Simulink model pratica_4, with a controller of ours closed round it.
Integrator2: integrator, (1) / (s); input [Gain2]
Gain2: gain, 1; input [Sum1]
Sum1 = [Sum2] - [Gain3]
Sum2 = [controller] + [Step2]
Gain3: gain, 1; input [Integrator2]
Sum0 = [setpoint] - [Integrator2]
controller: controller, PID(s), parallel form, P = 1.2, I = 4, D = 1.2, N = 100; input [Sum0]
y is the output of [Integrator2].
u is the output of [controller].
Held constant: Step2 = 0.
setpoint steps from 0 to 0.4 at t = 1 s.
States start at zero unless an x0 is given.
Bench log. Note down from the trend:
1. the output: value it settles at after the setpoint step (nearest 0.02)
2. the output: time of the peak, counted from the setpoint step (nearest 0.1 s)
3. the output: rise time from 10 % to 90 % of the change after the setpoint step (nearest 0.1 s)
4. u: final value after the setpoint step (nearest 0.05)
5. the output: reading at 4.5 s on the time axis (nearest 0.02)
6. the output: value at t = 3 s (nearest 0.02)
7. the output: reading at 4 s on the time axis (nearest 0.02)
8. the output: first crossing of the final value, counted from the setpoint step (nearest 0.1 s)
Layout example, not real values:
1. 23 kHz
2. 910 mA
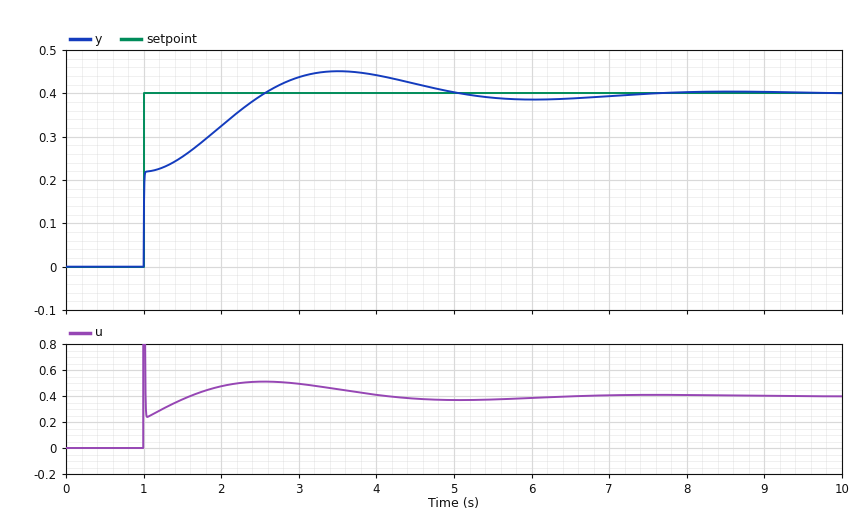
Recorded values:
1. 0.40
2. 2.5 s
3. 1.2 s
4. 0.40
5. 0.42
6. 0.44
7. 0.44
8. 1.6 s
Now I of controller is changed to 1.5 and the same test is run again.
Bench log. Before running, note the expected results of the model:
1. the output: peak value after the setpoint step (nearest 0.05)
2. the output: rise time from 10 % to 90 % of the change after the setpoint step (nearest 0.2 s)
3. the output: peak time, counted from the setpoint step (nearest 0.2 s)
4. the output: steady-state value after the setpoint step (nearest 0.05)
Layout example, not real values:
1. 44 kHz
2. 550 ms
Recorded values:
1. 0.40
2. 2.4 s
3. 4.8 s
4. 0.40
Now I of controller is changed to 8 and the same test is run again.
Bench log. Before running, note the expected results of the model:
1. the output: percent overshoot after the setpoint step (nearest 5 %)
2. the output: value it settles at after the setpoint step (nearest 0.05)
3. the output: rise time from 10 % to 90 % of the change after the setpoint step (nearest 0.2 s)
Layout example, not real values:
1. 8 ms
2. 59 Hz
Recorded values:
1. 20 %
2. 0.40
3. 0.8 s
